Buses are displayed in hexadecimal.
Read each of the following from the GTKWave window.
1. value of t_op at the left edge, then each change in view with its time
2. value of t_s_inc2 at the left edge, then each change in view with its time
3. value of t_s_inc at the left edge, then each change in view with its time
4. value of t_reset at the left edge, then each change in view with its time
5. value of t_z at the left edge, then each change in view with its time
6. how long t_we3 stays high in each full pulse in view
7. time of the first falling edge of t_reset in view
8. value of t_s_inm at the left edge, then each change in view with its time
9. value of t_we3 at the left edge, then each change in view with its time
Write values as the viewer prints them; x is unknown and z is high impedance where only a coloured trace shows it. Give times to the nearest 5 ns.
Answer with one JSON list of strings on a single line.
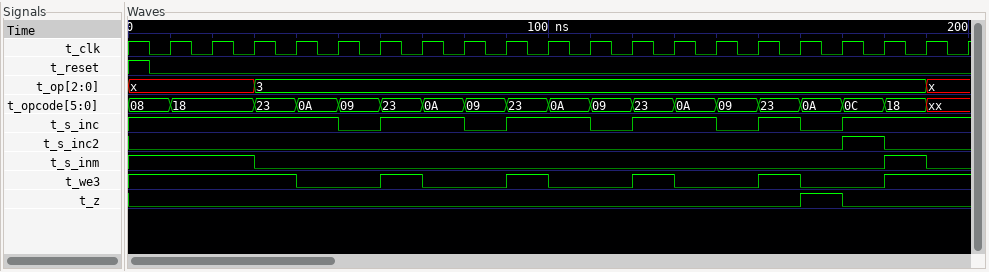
["x, 3 at 30 ns, x at 190 ns", "0, 1 at 170 ns, 0 at 180 ns", "1, 0 at 50 ns, 1 at 60 ns, 0 at 80 ns, 1 at 90 ns, 0 at 110 ns, 1 at 120 ns, 0 at 140 ns, 1 at 150 ns, 0 at 160 ns, 1 at 170 ns", "1, 0 at 5 ns", "0, 1 at 160 ns, 0 at 170 ns", "10 ns, 10 ns, 10 ns, 10 ns", "5 ns", "1, 0 at 30 ns, 1 at 180 ns, 0 at 190 ns", "1, 0 at 40 ns, 1 at 60 ns, 0 at 70 ns, 1 at 90 ns, 0 at 100 ns, 1 at 120 ns, 0 at 130 ns, 1 at 150 ns, 0 at 160 ns, 1 at 180 ns"]
